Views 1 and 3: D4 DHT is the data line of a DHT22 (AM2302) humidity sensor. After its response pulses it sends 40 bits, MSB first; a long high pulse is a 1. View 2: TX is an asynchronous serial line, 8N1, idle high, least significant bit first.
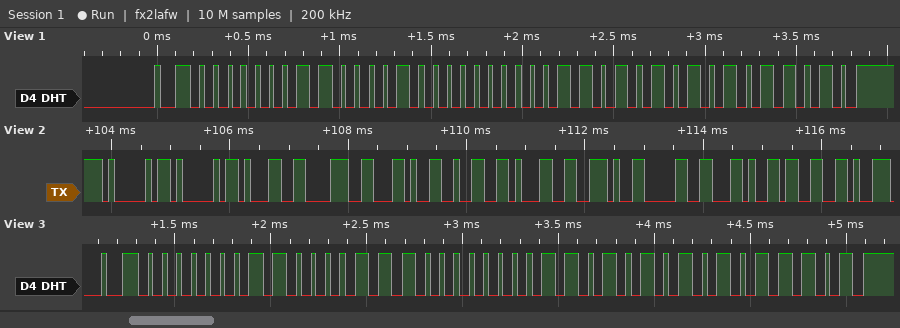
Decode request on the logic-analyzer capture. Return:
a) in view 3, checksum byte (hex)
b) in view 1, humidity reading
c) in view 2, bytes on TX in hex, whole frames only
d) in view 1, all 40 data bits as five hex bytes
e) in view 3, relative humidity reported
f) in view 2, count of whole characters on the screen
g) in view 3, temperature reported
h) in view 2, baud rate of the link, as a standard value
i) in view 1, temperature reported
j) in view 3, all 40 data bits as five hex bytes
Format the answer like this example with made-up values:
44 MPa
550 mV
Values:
0x5D
38.8 %
41 41 31 38 2C 32 31 2E 30 2C 33
01 84 00 D5 5A
39.1 %
11
21.3 °C
9600 baud
21.3 °C
01 87 00 D5 5D
